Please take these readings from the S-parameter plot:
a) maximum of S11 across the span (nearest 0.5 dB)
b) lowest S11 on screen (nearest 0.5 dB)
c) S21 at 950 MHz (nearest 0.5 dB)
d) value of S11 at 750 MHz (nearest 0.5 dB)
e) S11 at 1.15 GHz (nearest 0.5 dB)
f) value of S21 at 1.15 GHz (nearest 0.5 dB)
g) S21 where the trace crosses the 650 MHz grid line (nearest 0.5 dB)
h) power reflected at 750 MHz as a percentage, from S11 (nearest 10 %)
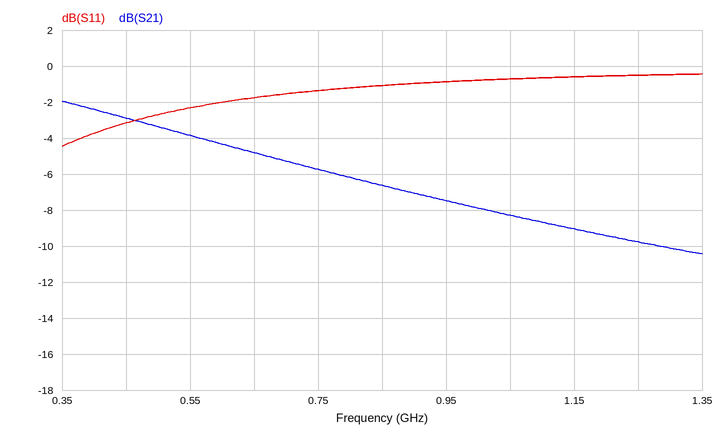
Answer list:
-0.5 dB
-4.5 dB
-7.5 dB
-1.5 dB
-0.5 dB
-9.0 dB
-5.0 dB
70 %
